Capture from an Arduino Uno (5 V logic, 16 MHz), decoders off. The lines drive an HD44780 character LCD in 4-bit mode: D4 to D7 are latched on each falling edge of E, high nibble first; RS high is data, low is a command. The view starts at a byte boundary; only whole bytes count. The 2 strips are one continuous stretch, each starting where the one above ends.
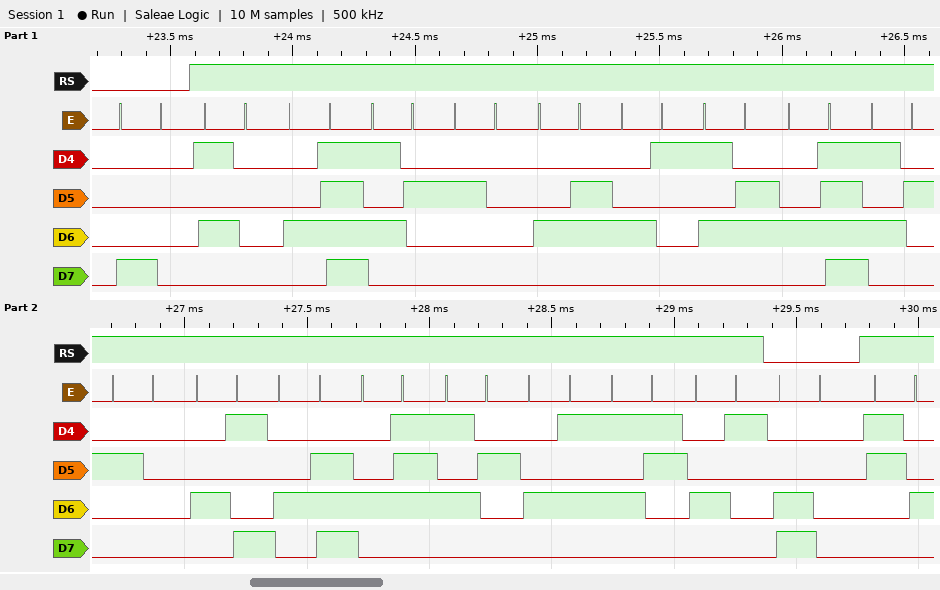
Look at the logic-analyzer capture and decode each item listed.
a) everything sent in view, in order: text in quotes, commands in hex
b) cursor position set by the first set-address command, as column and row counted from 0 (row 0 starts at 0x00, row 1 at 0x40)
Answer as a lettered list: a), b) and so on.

a) 0x80 "POR FAVOR INGRESA" 0xC0 "4"
b) column 0, row 0
